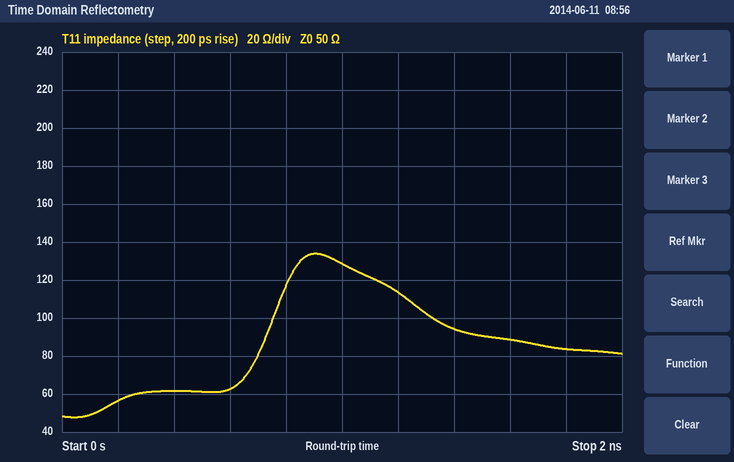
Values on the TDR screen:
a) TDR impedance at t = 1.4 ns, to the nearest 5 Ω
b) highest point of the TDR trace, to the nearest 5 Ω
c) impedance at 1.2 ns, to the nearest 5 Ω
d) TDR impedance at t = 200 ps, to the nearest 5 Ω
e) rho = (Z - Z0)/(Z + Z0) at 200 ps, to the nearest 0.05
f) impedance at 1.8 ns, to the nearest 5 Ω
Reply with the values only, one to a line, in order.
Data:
95 Ω
135 Ω
115 Ω
55 Ω
+0.05
85 Ω
